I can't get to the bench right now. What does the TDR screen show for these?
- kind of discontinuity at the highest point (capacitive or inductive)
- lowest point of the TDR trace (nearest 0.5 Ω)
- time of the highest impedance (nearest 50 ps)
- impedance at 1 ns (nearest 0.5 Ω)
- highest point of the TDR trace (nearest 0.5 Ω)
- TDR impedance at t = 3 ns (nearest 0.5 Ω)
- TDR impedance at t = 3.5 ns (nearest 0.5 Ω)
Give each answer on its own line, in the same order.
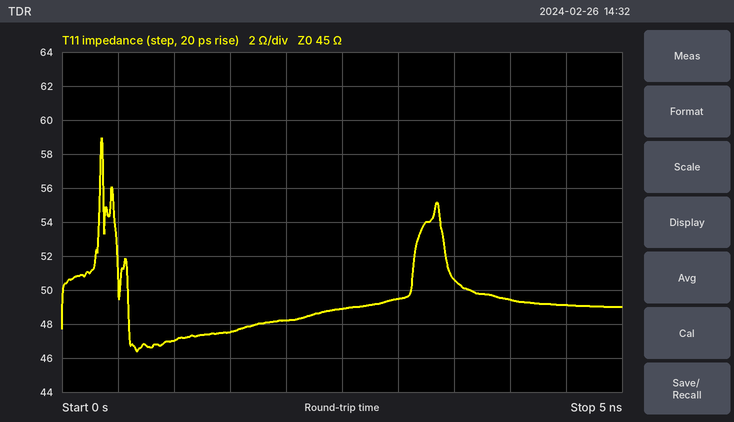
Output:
inductive
46.5 Ω
350 ps
47.0 Ω
59.0 Ω
49.5 Ω
50.5 Ω
